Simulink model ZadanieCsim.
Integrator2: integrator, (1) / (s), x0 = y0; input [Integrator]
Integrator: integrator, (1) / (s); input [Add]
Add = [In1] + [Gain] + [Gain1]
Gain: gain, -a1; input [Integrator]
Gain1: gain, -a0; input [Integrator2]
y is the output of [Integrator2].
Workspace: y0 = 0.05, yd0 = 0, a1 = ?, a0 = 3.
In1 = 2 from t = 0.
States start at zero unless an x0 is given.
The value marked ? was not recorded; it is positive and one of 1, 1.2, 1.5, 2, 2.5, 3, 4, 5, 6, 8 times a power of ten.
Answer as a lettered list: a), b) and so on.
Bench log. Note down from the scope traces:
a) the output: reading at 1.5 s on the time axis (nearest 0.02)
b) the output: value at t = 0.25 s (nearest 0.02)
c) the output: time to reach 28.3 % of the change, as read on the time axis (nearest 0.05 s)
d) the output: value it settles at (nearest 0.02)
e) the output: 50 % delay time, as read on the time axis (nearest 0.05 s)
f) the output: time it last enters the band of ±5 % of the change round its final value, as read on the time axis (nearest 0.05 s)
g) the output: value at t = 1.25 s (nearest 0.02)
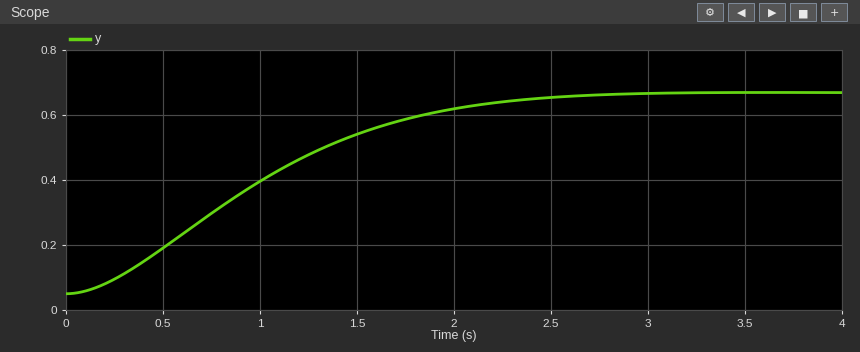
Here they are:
a) 0.54
b) 0.10
c) 0.60 s
d) 0.66
e) 0.90 s
f) 2.20 s
g) 0.48
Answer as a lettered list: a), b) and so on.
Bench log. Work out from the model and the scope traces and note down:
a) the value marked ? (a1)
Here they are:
a) 3
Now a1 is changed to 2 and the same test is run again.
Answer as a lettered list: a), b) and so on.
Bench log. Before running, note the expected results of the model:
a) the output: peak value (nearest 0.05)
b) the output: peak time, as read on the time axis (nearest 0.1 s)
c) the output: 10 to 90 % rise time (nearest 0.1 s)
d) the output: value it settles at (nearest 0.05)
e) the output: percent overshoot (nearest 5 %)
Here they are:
a) 0.75
b) 2.2 s
c) 1.0 s
d) 0.65
e) 10 %
